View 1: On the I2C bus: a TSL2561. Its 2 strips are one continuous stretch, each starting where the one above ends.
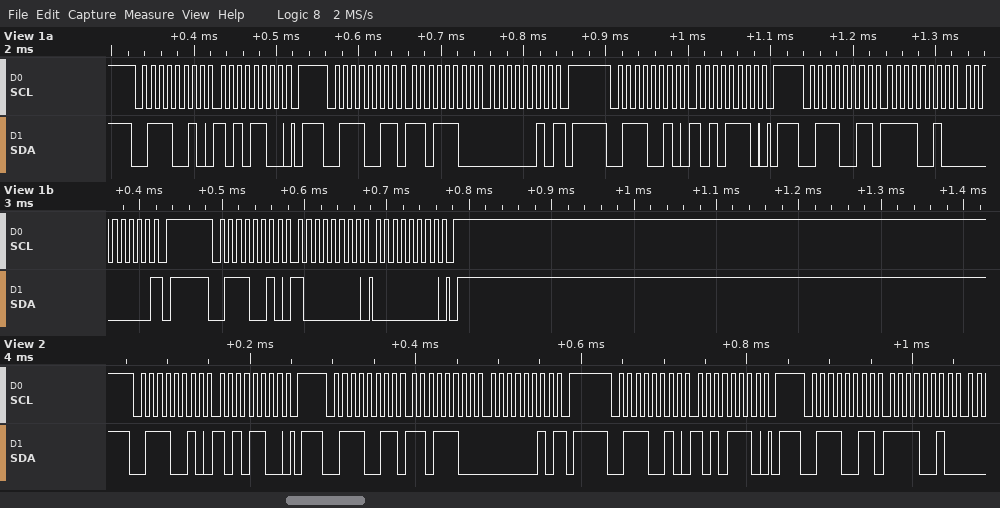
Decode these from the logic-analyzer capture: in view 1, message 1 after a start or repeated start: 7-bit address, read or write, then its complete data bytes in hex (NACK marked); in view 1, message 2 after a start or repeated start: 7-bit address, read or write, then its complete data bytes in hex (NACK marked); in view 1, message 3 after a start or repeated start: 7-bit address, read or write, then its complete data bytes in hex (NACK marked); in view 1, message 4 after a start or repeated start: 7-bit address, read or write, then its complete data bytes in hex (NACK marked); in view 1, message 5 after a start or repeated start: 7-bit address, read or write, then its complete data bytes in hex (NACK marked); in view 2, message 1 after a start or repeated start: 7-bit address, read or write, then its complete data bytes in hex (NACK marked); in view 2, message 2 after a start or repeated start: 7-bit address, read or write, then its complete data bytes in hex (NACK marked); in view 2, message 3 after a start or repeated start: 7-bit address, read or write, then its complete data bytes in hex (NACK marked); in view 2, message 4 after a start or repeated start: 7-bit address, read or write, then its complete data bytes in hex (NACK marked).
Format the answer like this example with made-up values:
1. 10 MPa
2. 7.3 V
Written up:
1. 0x39 write: AC
2. 0x39 read: DC 02 NACK
3. 0x39 write: AE
4. 0x39 read: F2 00 NACK
5. 0x39 write: 80 00
6. 0x39 write: AC
7. 0x39 read: DC 02 NACK
8. 0x39 write: AE
9. 0x39 read: F2
